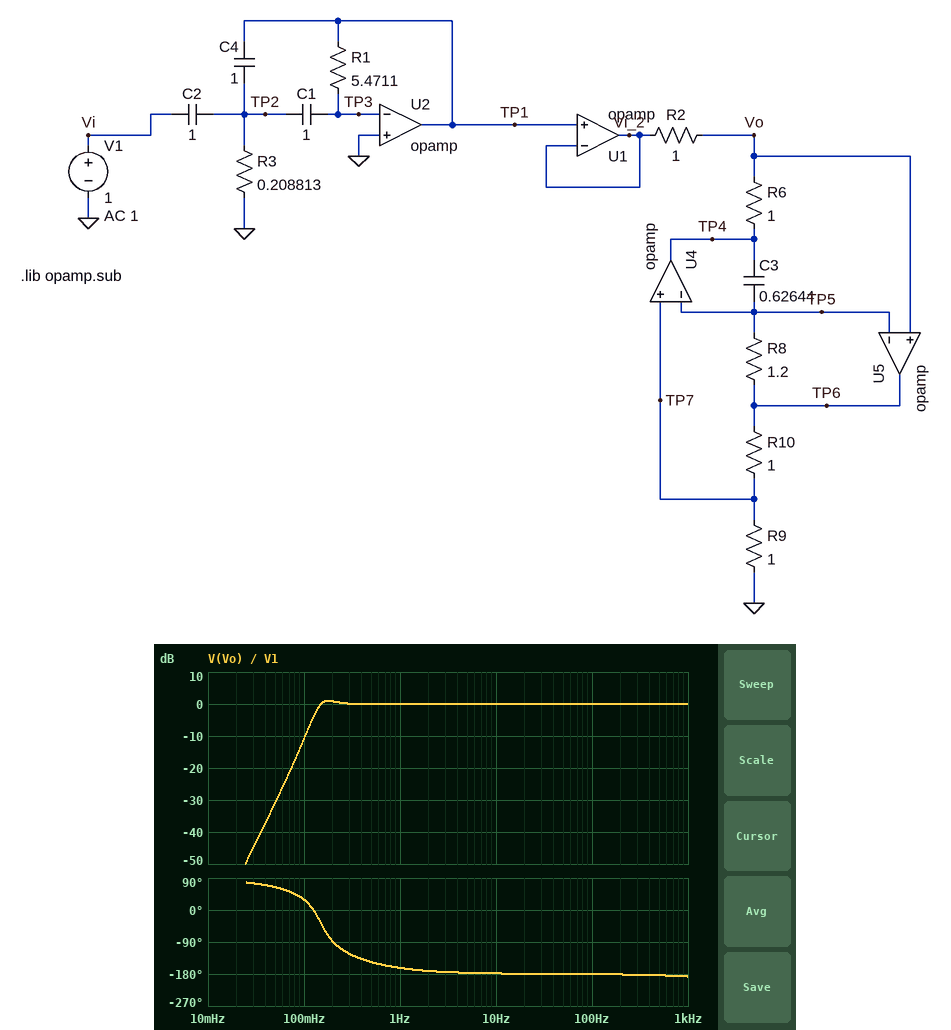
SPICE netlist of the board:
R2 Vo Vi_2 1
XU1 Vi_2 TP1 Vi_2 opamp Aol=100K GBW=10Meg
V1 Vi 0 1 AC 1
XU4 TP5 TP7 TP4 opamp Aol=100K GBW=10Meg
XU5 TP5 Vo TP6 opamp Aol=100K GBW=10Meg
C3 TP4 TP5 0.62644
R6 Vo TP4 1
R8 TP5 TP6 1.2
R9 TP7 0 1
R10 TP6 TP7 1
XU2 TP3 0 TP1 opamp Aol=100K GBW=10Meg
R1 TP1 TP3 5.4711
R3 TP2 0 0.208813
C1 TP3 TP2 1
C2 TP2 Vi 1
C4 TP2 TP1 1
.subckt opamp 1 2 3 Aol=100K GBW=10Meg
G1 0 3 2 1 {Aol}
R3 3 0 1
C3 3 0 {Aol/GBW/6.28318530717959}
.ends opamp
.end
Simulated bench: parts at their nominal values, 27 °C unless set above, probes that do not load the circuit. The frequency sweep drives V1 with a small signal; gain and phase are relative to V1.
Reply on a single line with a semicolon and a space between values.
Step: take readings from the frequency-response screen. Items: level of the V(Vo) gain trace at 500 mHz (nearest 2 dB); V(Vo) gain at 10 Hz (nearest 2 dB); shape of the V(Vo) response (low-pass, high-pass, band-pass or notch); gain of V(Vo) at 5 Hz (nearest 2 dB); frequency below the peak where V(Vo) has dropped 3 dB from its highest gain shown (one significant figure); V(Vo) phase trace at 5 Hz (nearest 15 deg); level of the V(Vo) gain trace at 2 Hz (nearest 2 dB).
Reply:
0 dB; 0 dB; high-pass; 0 dB; 100 mHz; -180 deg; 0 dB
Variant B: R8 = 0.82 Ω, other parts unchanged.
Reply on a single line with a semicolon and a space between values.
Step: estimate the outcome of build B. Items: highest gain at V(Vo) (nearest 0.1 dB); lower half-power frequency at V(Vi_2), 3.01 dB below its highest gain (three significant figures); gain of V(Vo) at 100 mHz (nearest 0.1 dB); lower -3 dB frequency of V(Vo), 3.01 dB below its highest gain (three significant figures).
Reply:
0 dB; 126 mHz; -13.8 dB; 146 mHz
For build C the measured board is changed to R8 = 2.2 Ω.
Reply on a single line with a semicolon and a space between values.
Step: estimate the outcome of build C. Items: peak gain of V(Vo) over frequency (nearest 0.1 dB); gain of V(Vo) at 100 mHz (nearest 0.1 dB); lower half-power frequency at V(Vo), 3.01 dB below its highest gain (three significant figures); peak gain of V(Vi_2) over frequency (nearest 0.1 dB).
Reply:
3.3 dB; -7.2 dB; 131 mHz; 5.0 dB
